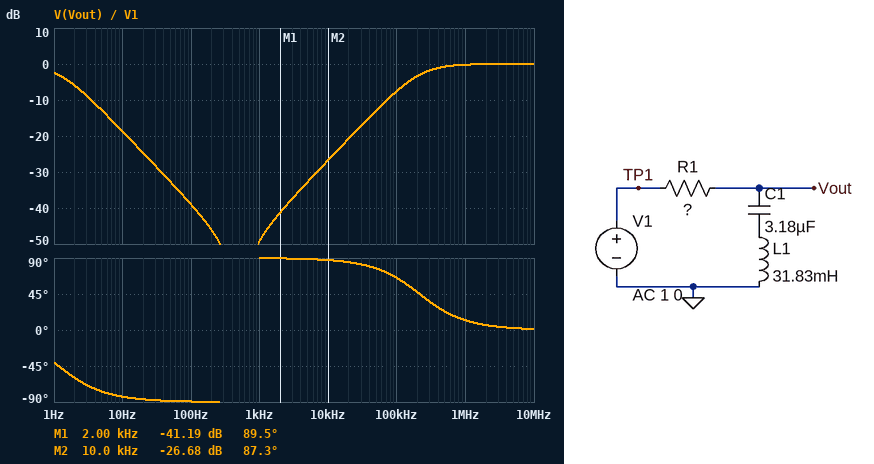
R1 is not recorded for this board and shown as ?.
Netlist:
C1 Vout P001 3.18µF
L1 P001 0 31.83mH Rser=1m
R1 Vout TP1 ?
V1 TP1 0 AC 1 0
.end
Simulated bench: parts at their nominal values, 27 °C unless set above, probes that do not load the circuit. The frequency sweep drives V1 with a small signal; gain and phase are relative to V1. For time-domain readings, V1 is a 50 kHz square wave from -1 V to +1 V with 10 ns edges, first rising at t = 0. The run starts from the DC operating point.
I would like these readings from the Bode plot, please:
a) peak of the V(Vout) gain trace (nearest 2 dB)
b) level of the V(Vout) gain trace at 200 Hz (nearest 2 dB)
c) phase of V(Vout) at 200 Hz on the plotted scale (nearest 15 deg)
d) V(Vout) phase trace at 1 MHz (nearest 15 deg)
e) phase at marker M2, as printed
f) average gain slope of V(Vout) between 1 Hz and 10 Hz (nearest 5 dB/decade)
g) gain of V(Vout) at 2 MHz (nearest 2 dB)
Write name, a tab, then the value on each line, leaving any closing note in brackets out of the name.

peak of the V(Vout) gain trace	0 dB
level of the V(Vout) gain trace at 200 Hz	-46 dB
phase of V(Vout) at 200 Hz on the plotted scale	-90 deg
V(Vout) phase trace at 1 MHz	15 deg
phase at marker M2, as printed	87.3 deg
average gain slope of V(Vout) between 1 Hz and 10 Hz	-15 dB/decade
gain of V(Vout) at 2 MHz	0 dB
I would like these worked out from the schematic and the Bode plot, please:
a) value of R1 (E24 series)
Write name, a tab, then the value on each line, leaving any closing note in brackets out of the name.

value of R1	43 kΩ
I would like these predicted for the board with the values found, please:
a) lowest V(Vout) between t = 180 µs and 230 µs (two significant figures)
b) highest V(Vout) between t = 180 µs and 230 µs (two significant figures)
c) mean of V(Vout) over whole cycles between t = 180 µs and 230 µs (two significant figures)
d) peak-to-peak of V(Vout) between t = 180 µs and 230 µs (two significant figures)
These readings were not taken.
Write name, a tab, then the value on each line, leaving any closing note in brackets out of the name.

lowest V(Vout) between t = 180 µs and 230 µs	-3.0 V
highest V(Vout) between t = 180 µs and 230 µs	990 mV
mean of V(Vout) over whole cycles between t = 180 µs and 230 µs	-1.0 V
peak-to-peak of V(Vout) between t = 180 µs and 230 µs	4.0 V
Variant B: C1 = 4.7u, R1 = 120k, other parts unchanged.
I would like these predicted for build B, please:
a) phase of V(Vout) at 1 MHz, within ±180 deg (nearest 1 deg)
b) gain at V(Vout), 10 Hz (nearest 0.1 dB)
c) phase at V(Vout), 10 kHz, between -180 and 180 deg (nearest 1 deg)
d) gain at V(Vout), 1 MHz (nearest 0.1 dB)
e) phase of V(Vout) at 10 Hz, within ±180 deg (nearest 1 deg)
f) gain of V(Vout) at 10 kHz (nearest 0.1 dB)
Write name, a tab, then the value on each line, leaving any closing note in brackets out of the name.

phase of V(Vout) at 1 MHz, within ±180 deg	31 deg
gain at V(Vout), 10 Hz	-31.0 dB
phase at V(Vout), 10 kHz, between -180 and 180 deg	89 deg
gain at V(Vout), 1 MHz	-1.3 dB
phase of V(Vout) at 10 Hz, within ±180 deg	-88 deg
gain of V(Vout) at 10 kHz	-35.6 dB
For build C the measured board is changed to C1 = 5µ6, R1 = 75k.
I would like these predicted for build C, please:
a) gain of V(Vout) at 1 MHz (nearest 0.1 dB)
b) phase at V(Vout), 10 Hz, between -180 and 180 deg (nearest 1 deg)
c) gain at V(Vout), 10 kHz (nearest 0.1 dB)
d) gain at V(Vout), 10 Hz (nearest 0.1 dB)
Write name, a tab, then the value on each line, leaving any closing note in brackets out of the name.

gain of V(Vout) at 1 MHz	-0.6 dB
phase at V(Vout), 10 Hz, between -180 and 180 deg	-88 deg
gain at V(Vout), 10 kHz	-31.5 dB
gain at V(Vout), 10 Hz	-28.4 dB
